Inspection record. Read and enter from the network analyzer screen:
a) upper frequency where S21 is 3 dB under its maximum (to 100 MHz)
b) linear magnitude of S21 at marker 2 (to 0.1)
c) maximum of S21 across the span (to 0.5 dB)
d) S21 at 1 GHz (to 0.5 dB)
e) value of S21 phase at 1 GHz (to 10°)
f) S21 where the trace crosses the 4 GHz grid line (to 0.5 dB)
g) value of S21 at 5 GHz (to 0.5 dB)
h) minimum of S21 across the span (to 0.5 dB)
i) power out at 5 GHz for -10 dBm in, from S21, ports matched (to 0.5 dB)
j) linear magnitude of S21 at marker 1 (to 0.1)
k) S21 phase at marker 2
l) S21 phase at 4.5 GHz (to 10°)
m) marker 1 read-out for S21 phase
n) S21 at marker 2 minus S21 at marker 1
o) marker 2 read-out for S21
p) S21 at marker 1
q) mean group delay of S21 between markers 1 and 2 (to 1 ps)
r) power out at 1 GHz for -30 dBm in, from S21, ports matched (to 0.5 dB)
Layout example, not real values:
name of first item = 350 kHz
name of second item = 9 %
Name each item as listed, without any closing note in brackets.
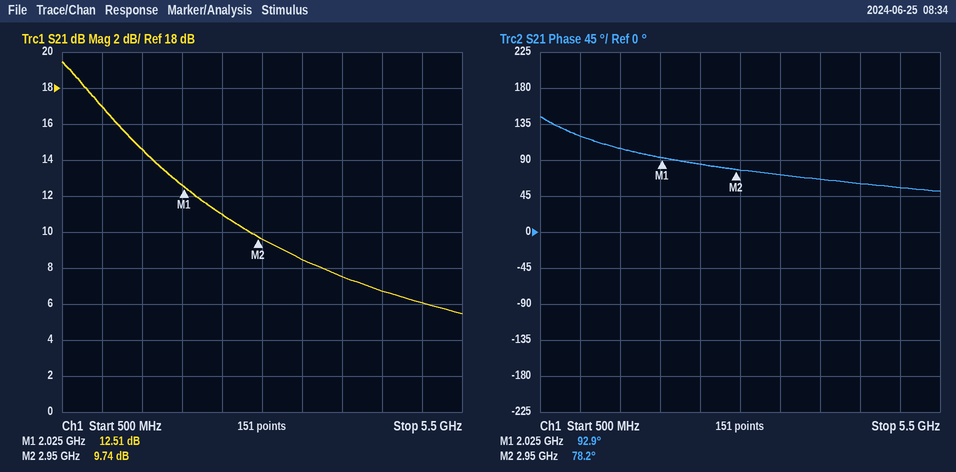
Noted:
upper frequency where S21 is 3 dB under its maximum = 1.1 GHz
linear magnitude of S21 at marker 2 = 3.1
maximum of S21 across the span = 19.5 dB
S21 at 1 GHz = 17.0 dB
value of S21 phase at 1 GHz = 120°
S21 where the trace crosses the 4 GHz grid line = 7.5 dB
value of S21 at 5 GHz = 6.0 dB
minimum of S21 across the span = 5.5 dB
power out at 5 GHz for -10 dBm in, from S21, ports matched = -4.0 dBm
linear magnitude of S21 at marker 1 = 4.2
S21 phase at marker 2 = 78.2°
S21 phase at 4.5 GHz = 60°
marker 1 read-out for S21 phase = 92.9°
S21 at marker 2 minus S21 at marker 1 = -2.77 dB
marker 2 read-out for S21 = 9.74 dB
S21 at marker 1 = 12.51 dB
mean group delay of S21 between markers 1 and 2 = 44 ps
power out at 1 GHz for -30 dBm in, from S21, ports matched = -13.0 dBm
